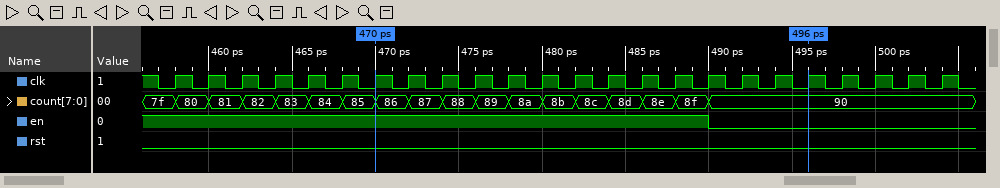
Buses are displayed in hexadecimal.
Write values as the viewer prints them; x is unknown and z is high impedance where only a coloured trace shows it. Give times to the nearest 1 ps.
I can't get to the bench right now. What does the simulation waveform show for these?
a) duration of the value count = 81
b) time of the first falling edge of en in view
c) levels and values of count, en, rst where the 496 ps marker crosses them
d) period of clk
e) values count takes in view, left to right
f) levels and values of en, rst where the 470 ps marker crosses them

2 ps
490 ps
count=90, en=0, rst=0
2 ps
7f, 80, 81, 82, 83, 84, 85, 86, 87, 88, 89, 8a, 8b, 8c, 8d, 8e, 8f, 90
en=1, rst=0
